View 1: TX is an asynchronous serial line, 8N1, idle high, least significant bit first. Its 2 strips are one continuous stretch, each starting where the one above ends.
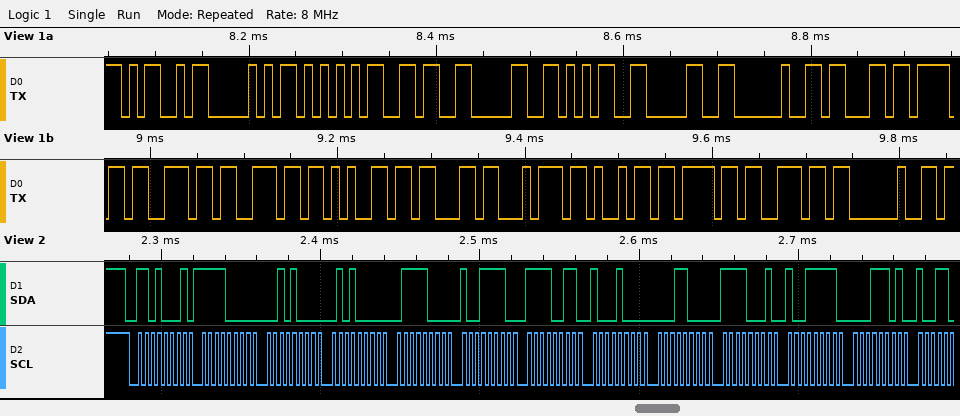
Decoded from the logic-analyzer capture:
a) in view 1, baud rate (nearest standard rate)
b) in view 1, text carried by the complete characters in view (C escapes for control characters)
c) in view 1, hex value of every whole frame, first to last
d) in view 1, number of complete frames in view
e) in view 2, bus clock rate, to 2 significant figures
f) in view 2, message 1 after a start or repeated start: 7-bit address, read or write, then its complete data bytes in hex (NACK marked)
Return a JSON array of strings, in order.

["115200 baud", "\"MPU6050 connection \"", "0x4D 0x50 0x55 0x36 0x30 0x35 0x30 0x20 0x63 0x6F 0x6E 0x6E 0x65 0x63 0x74 0x69 0x6F 0x6E 0x20", "19", "250 kHz", "0x68 read: F0 28 50 78 9E F3 88 18 F1 9F 1D"]
